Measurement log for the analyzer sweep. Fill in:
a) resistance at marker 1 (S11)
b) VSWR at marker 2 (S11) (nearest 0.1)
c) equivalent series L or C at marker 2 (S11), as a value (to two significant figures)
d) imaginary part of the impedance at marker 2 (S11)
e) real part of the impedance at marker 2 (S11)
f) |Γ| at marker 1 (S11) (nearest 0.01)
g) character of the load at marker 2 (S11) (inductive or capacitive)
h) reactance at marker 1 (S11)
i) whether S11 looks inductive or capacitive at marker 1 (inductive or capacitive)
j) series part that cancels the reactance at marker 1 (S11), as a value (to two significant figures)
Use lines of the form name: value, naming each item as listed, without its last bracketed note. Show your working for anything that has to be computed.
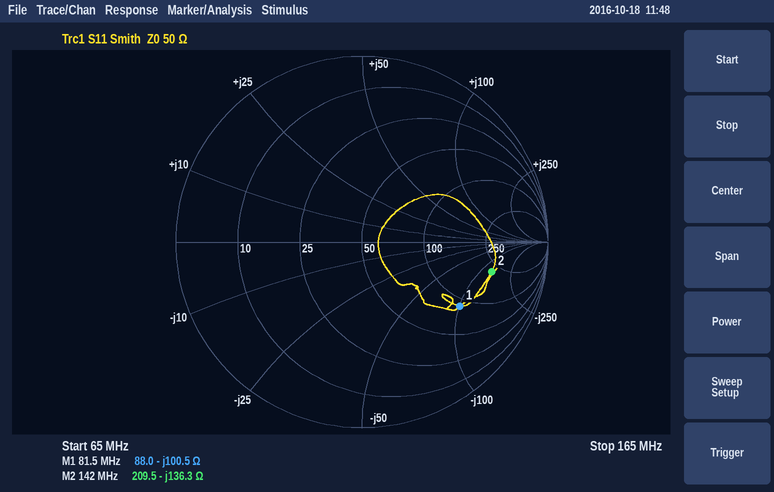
resistance at marker 1: 88.0 Ω
VSWR at marker 2 (S11): 6.0
equivalent series L or C at marker 2 (S11), as a value: C = 1/(2π × 142 MHz × 136.3 Ω) ≈ 8.2 pF
imaginary part of the impedance at marker 2: -136.3 Ω
real part of the impedance at marker 2: 209.5 Ω
|Γ| at marker 1 (S11): 0.63
character of the load at marker 2 (S11): capacitive
reactance at marker 1: -100.5 Ω
whether S11 looks inductive or capacitive at marker 1: capacitive
series part that cancels the reactance at marker 1 (S11), as a value: L = 100.5 Ω/(2π × 81.5 MHz) ≈ 196 nH, so 200 nH to two significant figures
